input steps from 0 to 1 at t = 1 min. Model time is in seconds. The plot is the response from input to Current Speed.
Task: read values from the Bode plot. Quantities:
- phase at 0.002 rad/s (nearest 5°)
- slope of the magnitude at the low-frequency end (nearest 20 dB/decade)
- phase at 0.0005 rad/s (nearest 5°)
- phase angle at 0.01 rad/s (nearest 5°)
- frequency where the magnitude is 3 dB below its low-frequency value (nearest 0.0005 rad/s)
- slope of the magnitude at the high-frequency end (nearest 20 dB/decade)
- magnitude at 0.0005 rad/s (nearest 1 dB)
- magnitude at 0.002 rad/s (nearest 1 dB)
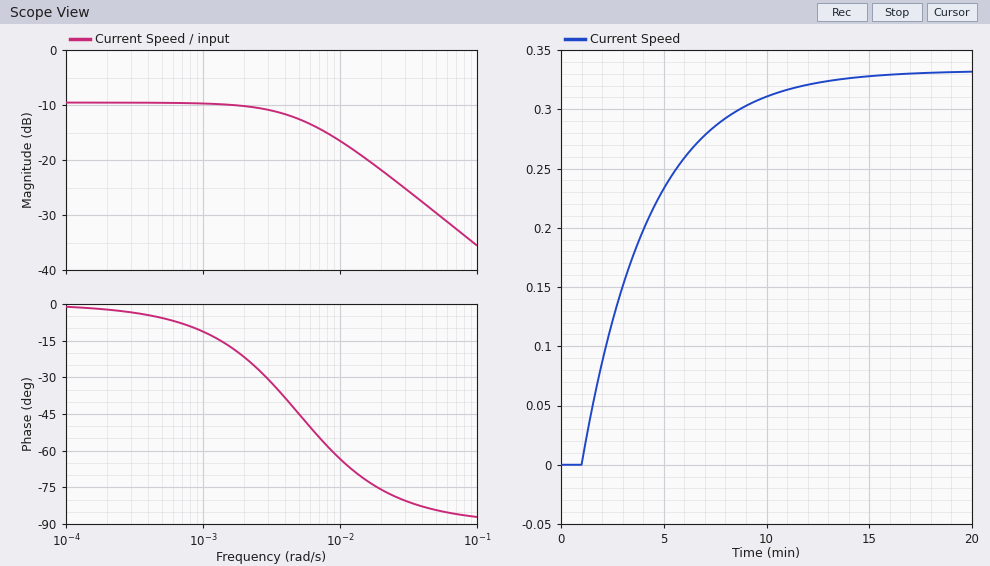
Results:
-20°
0 dB/decade
-5°
-65°
0.0050 rad/s
-20 dB/decade
-10 dB
-10 dB
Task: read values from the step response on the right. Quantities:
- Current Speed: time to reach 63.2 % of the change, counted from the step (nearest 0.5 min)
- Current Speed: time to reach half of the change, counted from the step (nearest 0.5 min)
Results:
3.5 min
2.5 min
